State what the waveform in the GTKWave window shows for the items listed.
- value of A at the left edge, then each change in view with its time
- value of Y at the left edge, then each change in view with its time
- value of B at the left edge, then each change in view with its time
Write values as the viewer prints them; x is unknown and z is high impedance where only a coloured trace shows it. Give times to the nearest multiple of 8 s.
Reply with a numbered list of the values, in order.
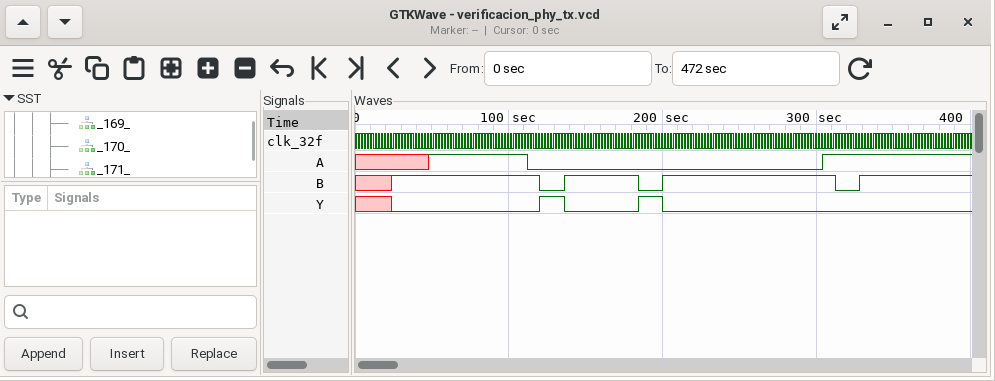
1. x, 1 at 48 s, 0 at 112 s, 1 at 304 s
2. x, 0 at 24 s, 1 at 120 s, 0 at 136 s, 1 at 184 s, 0 at 200 s
3. x, 1 at 24 s, 0 at 120 s, 1 at 136 s, 0 at 184 s, 1 at 200 s, 0 at 312 s, 1 at 328 s
